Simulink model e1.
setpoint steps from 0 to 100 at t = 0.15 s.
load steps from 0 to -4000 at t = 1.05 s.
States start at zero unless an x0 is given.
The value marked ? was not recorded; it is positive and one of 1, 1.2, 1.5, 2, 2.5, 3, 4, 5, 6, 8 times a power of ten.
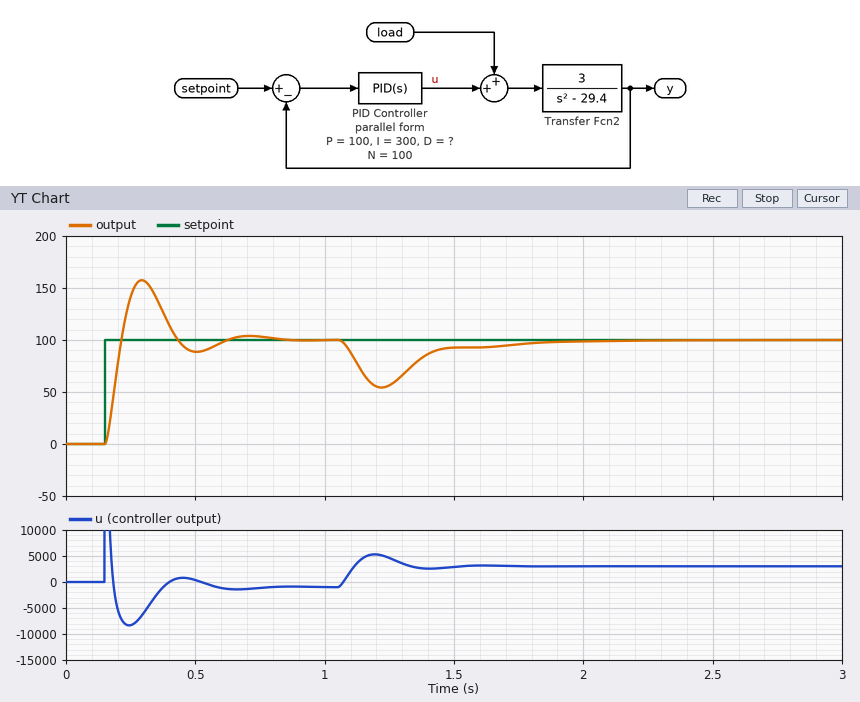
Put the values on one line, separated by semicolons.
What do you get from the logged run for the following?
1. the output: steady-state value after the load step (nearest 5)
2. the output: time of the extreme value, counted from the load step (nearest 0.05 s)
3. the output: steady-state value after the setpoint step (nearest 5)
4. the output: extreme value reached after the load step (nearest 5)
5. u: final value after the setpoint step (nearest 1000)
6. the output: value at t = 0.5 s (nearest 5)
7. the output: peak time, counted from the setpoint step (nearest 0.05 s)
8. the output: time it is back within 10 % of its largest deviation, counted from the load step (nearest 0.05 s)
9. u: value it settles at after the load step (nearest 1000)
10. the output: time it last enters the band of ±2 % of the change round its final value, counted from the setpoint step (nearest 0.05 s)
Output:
100; 0.15 s; 100; 55; -1000; 90; 0.15 s; 0.70 s; 3000; 0.65 s
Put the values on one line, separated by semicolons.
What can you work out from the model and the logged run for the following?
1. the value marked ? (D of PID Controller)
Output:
5
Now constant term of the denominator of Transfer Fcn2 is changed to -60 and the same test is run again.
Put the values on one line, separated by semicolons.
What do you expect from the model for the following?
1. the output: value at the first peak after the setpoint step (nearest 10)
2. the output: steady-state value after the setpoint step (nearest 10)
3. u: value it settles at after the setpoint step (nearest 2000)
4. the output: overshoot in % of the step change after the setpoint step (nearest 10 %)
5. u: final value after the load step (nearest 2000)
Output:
170; 100; -2000; 70 %; 2000
